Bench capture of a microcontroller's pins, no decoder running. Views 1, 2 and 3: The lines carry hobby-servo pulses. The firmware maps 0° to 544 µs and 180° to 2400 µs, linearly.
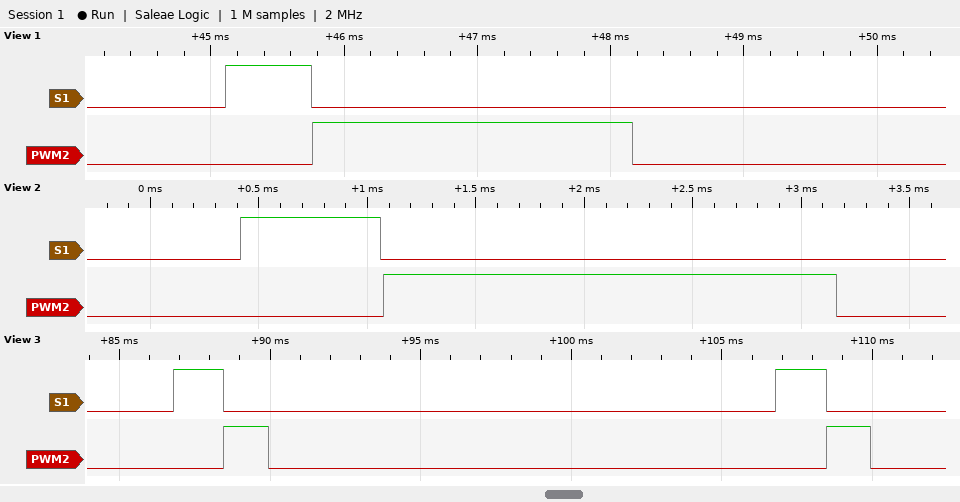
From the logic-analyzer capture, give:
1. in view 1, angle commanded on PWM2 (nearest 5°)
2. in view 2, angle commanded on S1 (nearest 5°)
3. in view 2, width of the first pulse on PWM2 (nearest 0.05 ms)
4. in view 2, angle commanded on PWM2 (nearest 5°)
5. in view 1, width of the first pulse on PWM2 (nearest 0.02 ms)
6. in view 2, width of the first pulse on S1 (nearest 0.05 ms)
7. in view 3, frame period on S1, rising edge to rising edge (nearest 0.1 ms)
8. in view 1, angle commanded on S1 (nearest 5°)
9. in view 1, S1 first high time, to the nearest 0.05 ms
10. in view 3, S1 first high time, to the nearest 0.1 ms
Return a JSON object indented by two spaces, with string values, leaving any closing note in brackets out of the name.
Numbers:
{
  "in view 1, angle commanded on PWM2": "180°",
  "in view 2, angle commanded on S1": "10°",
  "in view 2, width of the first pulse on PWM2": "2.10 ms",
  "in view 2, angle commanded on PWM2": "150°",
  "in view 1, width of the first pulse on PWM2": "2.40 ms",
  "in view 2, width of the first pulse on S1": "0.65 ms",
  "in view 3, frame period on S1, rising edge to rising edge": "20.0 ms",
  "in view 1, angle commanded on S1": "10°",
  "in view 1, S1 first high time, to the nearest 0.05 ms": "0.65 ms",
  "in view 3, S1 first high time, to the nearest 0.1 ms": "1.7 ms"
}
